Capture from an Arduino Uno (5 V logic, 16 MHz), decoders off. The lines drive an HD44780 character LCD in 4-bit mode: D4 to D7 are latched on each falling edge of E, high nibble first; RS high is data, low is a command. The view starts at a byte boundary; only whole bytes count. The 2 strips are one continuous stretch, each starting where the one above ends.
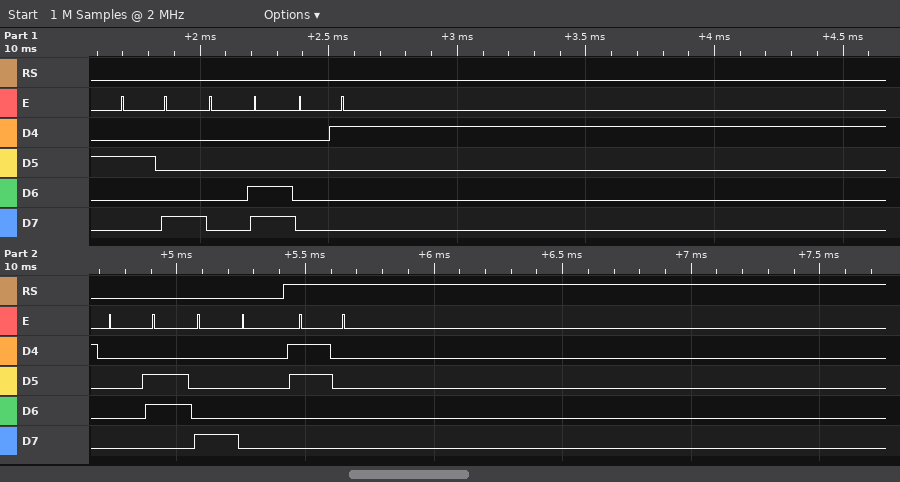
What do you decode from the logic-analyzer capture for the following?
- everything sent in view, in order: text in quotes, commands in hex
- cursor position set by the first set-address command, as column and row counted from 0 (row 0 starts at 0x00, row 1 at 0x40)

0x28 0x0C 0x01 0x06 0x80 "0"
column 0, row 0
